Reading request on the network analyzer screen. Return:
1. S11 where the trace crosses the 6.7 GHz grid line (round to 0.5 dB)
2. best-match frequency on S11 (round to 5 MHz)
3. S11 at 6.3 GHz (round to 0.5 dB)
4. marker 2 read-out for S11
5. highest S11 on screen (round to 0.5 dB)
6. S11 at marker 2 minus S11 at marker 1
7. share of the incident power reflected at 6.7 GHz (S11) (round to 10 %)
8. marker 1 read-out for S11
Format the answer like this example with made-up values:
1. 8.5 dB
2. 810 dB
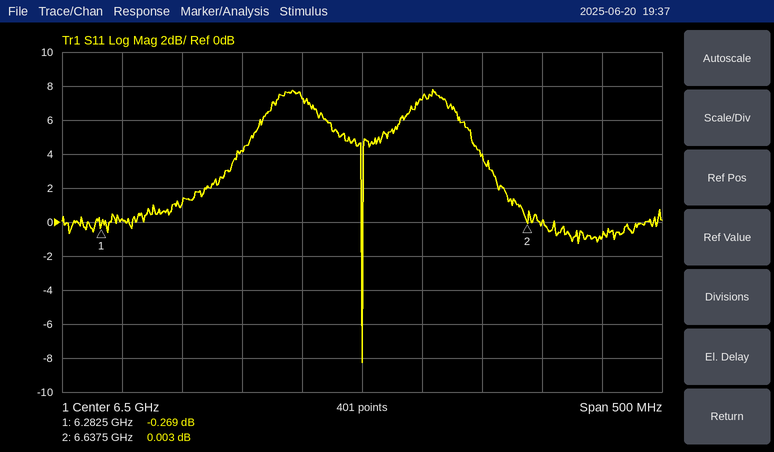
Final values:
1. -1.0 dB
2. 6.500 GHz
3. 0.0 dB
4. 0.003 dB
5. 8.0 dB
6. 0.272 dB
7. 80 %
8. -0.269 dB
